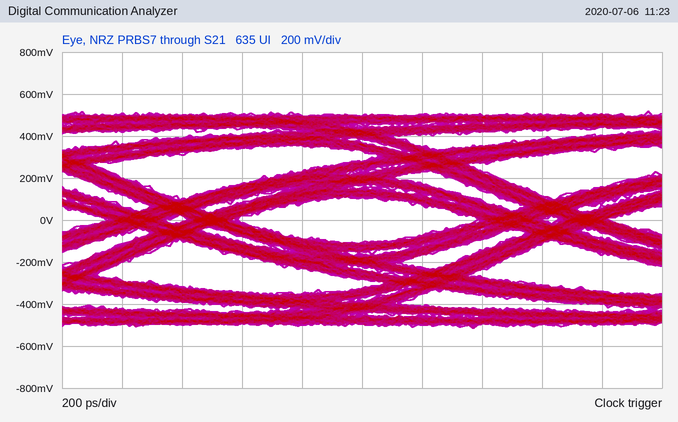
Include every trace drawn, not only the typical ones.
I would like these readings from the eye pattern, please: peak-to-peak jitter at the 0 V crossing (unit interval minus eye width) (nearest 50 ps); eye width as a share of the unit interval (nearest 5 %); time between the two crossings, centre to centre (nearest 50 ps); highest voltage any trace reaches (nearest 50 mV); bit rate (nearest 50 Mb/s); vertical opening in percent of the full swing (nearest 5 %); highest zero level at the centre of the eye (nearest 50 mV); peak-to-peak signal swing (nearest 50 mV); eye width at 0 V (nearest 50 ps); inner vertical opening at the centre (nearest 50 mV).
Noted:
450 ps
65 %
1.25 ns
500 mV
800 Mb/s
20 %
-100 mV
1.05 V
800 ps
200 mV
